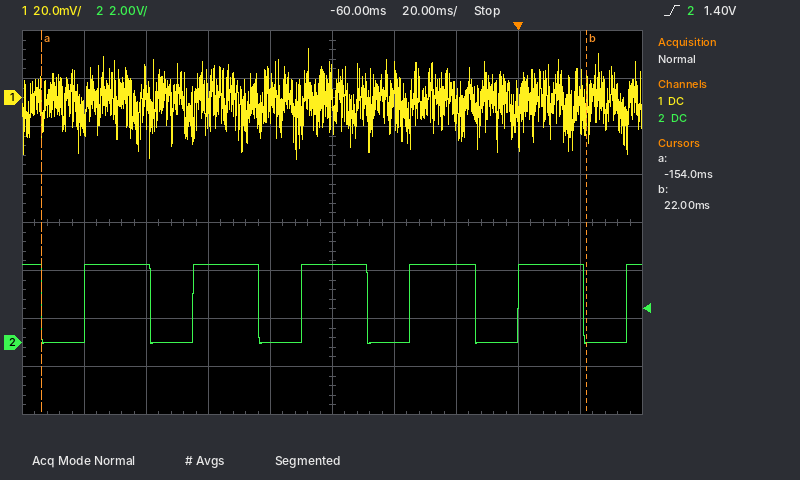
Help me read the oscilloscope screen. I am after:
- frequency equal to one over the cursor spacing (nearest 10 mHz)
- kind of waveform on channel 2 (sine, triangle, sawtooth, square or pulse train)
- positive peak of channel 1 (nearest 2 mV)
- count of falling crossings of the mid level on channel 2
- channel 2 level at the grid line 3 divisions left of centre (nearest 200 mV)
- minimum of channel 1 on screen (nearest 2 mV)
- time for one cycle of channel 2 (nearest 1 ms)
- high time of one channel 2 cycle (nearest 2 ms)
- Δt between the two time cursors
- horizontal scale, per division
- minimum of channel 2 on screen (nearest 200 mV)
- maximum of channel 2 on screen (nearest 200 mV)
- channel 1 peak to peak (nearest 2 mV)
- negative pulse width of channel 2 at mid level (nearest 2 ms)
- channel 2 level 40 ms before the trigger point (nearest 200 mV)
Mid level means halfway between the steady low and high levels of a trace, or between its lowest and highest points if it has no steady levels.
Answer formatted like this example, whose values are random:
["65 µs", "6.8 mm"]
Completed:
["5.68 Hz", "pulse train", "20 mV", "6", "3.2 V", "-26 mV", "35 ms", "22 ms", "176 ms", "20 ms", "0.0 V", "3.2 V", "46 mV", "14 ms", "0.0 V"]
